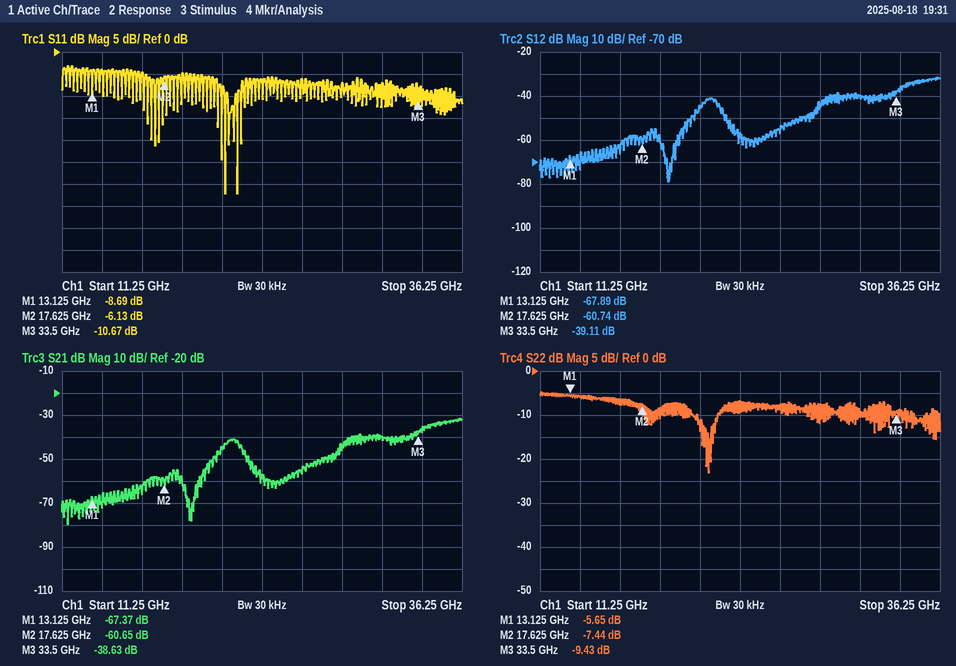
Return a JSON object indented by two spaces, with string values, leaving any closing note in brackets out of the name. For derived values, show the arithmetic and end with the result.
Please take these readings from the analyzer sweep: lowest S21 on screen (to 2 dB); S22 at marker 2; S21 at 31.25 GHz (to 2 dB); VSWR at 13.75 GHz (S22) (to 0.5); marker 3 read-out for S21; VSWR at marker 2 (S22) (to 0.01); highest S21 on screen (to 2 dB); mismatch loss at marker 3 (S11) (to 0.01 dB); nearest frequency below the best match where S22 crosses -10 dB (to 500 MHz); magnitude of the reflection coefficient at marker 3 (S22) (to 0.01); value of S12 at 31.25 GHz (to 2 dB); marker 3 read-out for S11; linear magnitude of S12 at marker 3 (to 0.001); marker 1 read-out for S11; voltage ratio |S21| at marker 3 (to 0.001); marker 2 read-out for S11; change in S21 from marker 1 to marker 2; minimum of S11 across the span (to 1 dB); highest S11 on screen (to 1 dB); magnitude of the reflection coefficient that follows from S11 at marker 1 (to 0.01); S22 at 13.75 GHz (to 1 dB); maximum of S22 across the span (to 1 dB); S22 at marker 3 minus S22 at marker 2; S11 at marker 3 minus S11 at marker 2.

{
  "lowest S21 on screen": "-80 dB",
  "S22 at marker 2": "-7.44 dB",
  "S21 at 31.25 GHz": "-40 dB",
  "VSWR at 13.75 GHz (S22)": "|Γ| = 10^(-6/20) = 0.5012; VSWR = (1 + 0.5012)/(1 − 0.5012) ≈ 3.0",
  "marker 3 read-out for S21": "-38.63 dB",
  "VSWR at marker 2 (S22)": "(1 + 0.4246)/(1 − 0.4246) ≈ 2.48",
  "highest S21 on screen": "-32 dB",
  "mismatch loss at marker 3 (S11)": "−10 log10(1 − 10^(-10.67/10)) ≈ 0.39 dB",
  "nearest frequency below the best match where S22 crosses -10 dB": "21.0 GHz",
  "magnitude of the reflection coefficient at marker 3 (S22)": "10^(-9.43/20) ≈ 0.34",
  "value of S12 at 31.25 GHz": "-40 dB",
  "marker 3 read-out for S11": "-10.67 dB",
  "linear magnitude of S12 at marker 3": "10^(-39.11/20) ≈ 0.011",
  "marker 1 read-out for S11": "-8.69 dB",
  "voltage ratio |S21| at marker 3": "10^(-38.63/20) ≈ 0.012",
  "marker 2 read-out for S11": "-6.13 dB",
  "change in S21 from marker 1 to marker 2": "-60.65 − (-67.37) = 6.72 dB",
  "minimum of S11 across the span": "-32 dB",
  "highest S11 on screen": "-3 dB",
  "magnitude of the reflection coefficient that follows from S11 at marker 1": "10^(-8.69/20) ≈ 0.37",
  "S22 at 13.75 GHz": "-6 dB",
  "maximum of S22 across the span": "-5 dB",
  "S22 at marker 3 minus S22 at marker 2": "-9.43 − (-7.44) = -1.99 dB",
  "S11 at marker 3 minus S11 at marker 2": "-10.67 − (-6.13) = -4.54 dB"
}
